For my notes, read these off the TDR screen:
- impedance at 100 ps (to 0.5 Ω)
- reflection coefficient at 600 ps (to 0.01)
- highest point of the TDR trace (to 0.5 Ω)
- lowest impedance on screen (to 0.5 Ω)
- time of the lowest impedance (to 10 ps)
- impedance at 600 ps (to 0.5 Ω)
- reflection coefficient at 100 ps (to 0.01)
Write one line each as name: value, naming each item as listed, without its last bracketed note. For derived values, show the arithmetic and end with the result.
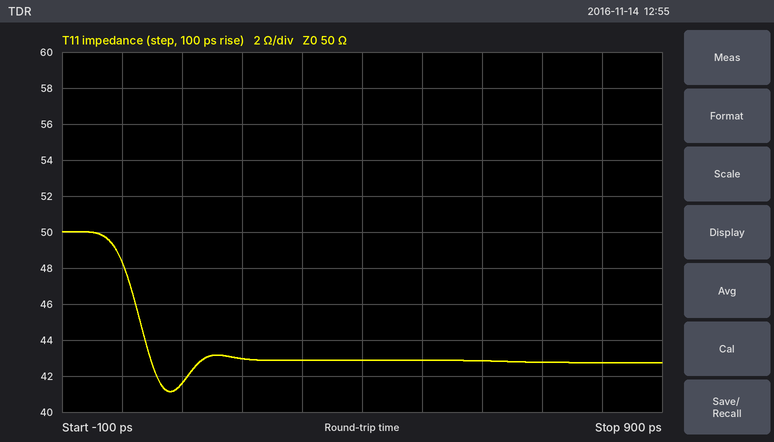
impedance at 100 ps: 41.5 Ω
reflection coefficient at 600 ps: (43 − 50)/(43 + 50) ≈ -0.08
highest point of the TDR trace: 50.0 Ω
lowest impedance on screen: 41.0 Ω
time of the lowest impedance: 80 ps
impedance at 600 ps: 43.0 Ω
reflection coefficient at 100 ps: (41.5 − 50)/(41.5 + 50) ≈ -0.09
